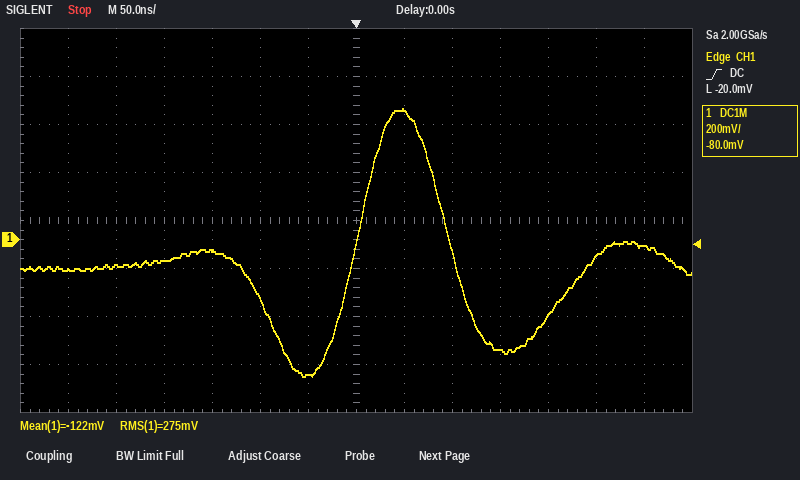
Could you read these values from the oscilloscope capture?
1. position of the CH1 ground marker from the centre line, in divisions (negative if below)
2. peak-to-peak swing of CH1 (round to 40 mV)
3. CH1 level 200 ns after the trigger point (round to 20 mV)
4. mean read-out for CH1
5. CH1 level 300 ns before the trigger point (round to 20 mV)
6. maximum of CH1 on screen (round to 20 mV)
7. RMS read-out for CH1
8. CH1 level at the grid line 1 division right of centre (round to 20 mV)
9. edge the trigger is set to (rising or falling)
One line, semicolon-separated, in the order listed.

-0.4 div; 1.12 V; -320 mV; -122 mV; -120 mV; 540 mV; 275 mV; 540 mV; rising
